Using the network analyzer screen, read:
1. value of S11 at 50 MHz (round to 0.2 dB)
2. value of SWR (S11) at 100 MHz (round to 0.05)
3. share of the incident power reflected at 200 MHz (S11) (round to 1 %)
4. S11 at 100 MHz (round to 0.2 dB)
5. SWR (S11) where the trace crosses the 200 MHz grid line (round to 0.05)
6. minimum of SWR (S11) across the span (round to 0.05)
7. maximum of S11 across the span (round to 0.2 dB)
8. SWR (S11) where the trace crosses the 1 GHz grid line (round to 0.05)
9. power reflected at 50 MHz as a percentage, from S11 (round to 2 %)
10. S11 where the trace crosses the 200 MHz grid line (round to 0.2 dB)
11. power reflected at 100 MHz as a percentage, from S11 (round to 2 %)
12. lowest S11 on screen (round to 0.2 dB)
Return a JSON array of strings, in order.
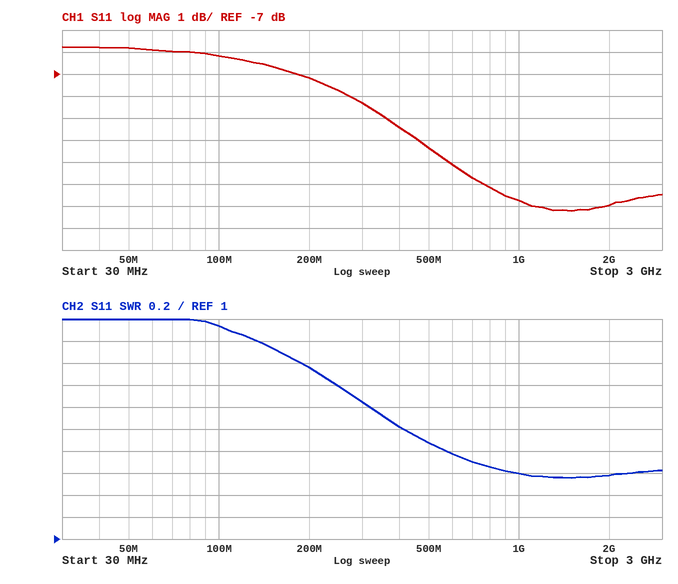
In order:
["-5.8 dB", "2.95", "19 %", "-6.2 dB", "2.55", "1.55", "-5.8 dB", "1.60", "26 %", "-7.2 dB", "24 %", "-13.2 dB"]
